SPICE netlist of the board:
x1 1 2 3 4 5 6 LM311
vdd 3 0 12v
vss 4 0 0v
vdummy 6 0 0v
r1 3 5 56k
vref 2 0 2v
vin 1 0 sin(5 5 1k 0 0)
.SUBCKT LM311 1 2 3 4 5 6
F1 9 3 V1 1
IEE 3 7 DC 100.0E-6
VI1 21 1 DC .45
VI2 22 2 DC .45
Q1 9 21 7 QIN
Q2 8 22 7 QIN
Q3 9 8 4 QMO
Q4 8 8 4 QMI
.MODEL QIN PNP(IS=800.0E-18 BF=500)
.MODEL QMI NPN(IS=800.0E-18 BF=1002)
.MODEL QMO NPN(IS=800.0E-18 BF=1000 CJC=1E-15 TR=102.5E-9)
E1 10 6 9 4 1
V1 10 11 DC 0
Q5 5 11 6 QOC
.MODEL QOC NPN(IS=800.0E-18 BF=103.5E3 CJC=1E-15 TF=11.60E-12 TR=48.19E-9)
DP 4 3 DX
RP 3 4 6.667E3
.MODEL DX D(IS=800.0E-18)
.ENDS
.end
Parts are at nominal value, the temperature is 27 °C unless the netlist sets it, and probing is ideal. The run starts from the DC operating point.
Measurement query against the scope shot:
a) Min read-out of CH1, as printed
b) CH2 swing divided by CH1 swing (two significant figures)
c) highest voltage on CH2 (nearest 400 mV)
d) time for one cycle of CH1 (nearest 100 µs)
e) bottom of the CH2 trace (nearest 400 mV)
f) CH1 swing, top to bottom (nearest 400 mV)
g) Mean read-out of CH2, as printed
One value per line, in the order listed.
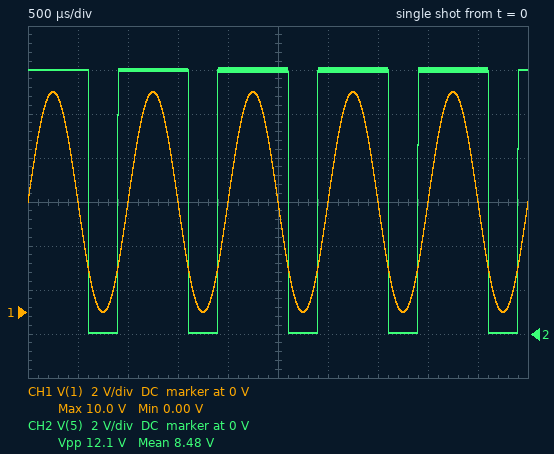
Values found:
0.00 V
1.2
12.0 V
1.0 ms
0 V
10.0 V
8.48 V
